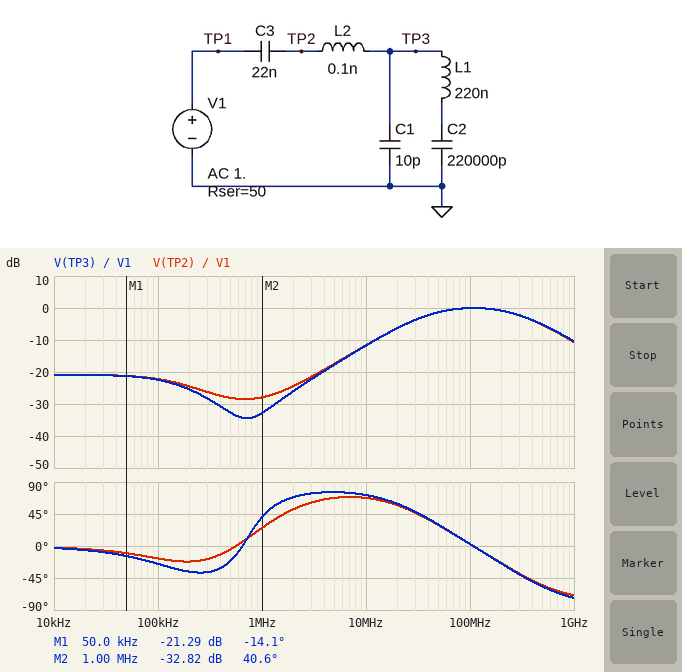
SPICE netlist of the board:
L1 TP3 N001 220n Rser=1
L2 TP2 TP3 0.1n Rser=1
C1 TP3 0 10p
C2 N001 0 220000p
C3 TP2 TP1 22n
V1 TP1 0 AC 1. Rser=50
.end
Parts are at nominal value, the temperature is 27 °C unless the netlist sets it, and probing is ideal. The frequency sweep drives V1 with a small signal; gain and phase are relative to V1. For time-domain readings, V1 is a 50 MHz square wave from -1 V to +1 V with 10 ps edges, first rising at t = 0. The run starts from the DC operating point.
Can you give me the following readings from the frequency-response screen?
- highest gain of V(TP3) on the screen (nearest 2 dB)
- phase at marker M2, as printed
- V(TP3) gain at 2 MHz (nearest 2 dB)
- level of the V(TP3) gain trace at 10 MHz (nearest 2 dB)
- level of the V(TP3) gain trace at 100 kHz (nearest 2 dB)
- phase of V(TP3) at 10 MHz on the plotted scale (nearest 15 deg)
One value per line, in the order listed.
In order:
0 dB
40.6 deg
-26 dB
-12 dB
-22 dB
75 deg
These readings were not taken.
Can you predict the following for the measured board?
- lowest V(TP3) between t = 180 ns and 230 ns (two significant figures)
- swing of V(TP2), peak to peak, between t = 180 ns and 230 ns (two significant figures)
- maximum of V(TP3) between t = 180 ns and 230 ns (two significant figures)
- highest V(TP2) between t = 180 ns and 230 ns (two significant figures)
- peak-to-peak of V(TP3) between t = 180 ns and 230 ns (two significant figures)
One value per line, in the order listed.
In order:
-1.5 V
3.0 V
1.5 V
1.5 V
3.0 V
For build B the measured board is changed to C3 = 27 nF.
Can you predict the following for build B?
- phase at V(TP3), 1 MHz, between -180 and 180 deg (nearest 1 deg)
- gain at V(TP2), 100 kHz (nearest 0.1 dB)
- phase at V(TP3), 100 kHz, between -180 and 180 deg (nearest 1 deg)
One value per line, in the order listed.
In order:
39 deg
-21.1 dB
-30 deg
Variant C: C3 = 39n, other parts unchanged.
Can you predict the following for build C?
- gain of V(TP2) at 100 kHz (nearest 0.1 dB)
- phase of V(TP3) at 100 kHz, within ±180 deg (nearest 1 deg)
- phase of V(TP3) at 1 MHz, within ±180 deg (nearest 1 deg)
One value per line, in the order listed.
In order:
-19.6 dB
-39 deg
37 deg
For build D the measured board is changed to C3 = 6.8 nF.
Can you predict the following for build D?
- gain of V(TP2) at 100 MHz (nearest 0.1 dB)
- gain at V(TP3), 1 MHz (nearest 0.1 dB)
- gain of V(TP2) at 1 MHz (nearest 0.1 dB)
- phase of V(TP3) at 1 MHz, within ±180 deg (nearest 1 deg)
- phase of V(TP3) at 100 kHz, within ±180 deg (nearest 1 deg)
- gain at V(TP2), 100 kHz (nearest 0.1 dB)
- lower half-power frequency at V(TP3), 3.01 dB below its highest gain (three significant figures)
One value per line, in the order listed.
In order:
0 dB
-33.5 dB
-28.6 dB
57 deg
-4 deg
-30.5 dB
33.5 MHz
